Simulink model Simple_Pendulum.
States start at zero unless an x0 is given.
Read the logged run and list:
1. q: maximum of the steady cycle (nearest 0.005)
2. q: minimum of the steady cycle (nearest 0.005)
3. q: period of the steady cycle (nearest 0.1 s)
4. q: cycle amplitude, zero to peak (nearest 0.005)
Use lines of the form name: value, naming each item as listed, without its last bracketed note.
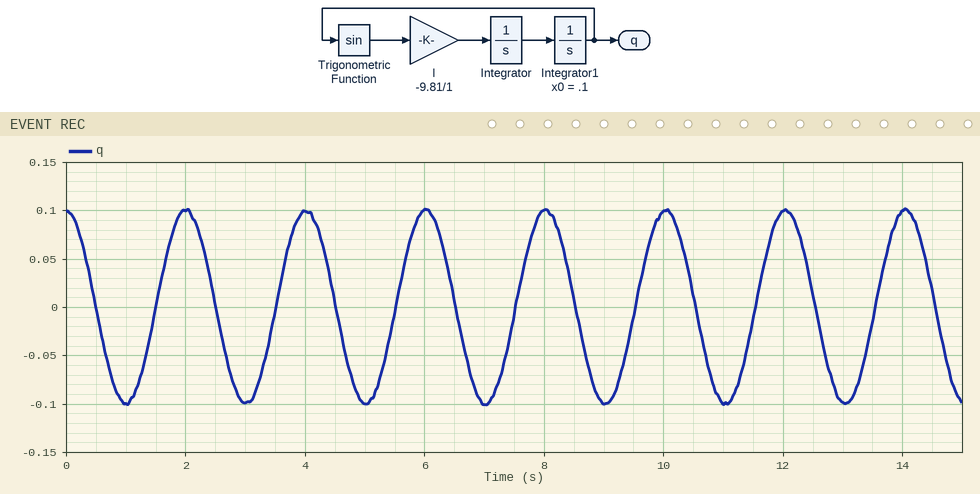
q: maximum of the steady cycle: 0.100
q: minimum of the steady cycle: -0.100
q: period of the steady cycle: 2.0 s
q: cycle amplitude, zero to peak: 0.100
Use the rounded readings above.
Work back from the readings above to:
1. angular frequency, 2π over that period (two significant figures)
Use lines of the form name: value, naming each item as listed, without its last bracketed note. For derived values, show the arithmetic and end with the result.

angular frequency, 2π over that period: 2π / 2 = 3.1 rad/s
